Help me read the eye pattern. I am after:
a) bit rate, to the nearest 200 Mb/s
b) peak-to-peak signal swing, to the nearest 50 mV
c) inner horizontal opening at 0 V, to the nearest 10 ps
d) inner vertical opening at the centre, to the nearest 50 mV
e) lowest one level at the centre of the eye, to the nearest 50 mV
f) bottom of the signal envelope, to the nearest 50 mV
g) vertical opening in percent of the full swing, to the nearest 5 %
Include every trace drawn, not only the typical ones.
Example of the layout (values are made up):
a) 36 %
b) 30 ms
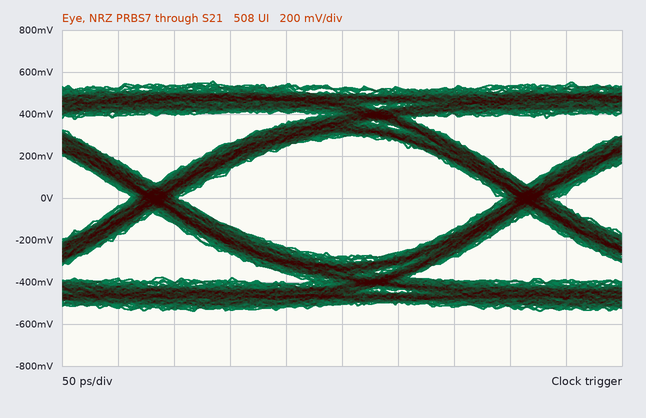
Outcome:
a) 3.0 Gb/s
b) 1.10 V
c) 290 ps
d) 550 mV
e) 300 mV
f) -550 mV
g) 50 %
